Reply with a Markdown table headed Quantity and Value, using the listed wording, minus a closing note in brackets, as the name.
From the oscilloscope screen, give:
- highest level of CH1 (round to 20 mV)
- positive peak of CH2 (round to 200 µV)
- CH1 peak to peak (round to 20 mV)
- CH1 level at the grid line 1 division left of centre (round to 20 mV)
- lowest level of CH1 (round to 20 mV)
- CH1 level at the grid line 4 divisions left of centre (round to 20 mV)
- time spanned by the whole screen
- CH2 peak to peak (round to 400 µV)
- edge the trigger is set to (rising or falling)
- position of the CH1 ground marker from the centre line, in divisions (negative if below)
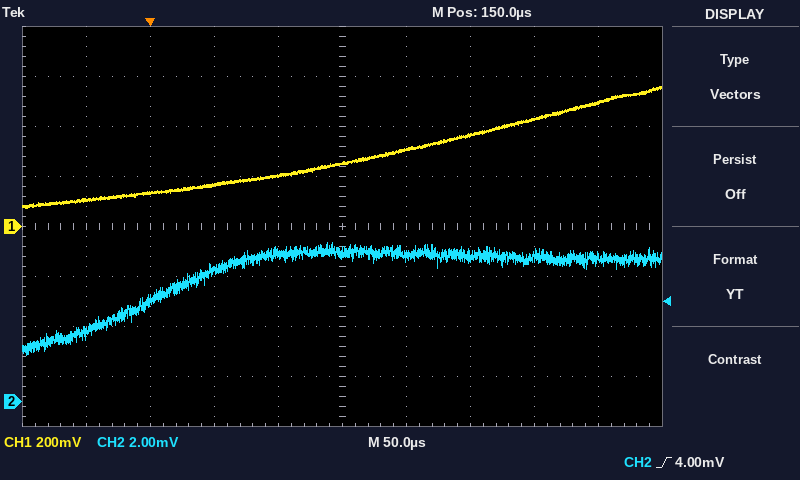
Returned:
| Quantity | Value |
|---|---|
| highest level of CH1 | 560 mV |
| positive peak of CH2 | 6.4 mV |
| CH1 peak to peak | 480 mV |
| CH1 level at the grid line 1 division left of centre | 200 mV |
| lowest level of CH1 | 80 mV |
| CH1 level at the grid line 4 divisions left of centre | 100 mV |
| time spanned by the whole screen | 500 µs |
| CH2 peak to peak | 4.4 mV |
| edge the trigger is set to | rising |
| position of the CH1 ground marker from the centre line, in divisions | 0.0 div |
